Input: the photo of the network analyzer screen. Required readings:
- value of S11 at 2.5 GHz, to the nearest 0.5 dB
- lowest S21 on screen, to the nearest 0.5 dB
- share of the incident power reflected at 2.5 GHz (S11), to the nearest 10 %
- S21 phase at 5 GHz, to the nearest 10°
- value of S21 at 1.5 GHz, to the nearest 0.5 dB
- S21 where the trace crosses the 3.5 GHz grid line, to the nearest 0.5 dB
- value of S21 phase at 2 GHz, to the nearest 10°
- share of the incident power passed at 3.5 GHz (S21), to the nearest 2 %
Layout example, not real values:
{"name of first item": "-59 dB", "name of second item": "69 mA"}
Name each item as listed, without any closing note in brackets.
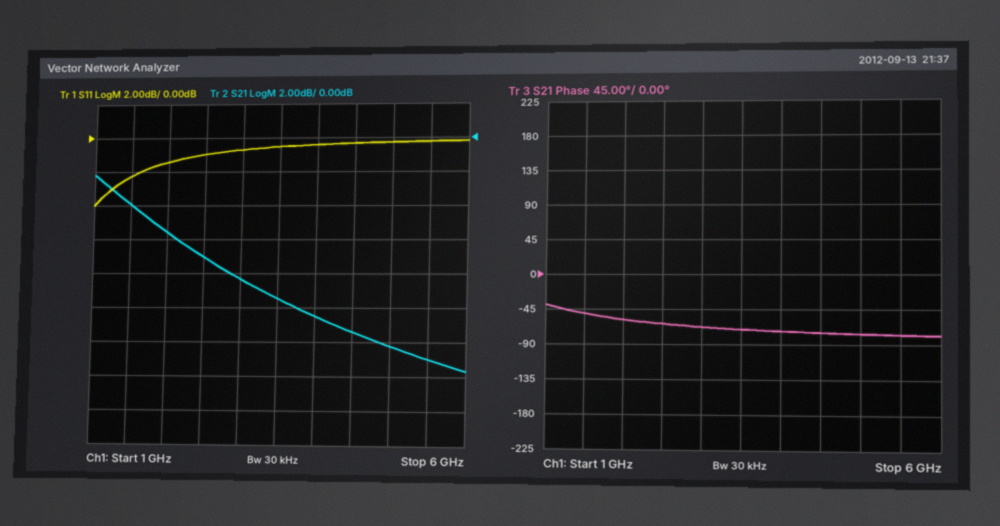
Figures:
{"value of S11 at 2.5 GHz, to the nearest 0.5 dB": "-1.0 dB", "lowest S21 on screen, to the nearest 0.5 dB": "-13.5 dB", "share of the incident power reflected at 2.5 GHz (S11), to the nearest 10 %": "80 %", "S21 phase at 5 GHz, to the nearest 10°": "-80°", "value of S21 at 1.5 GHz, to the nearest 0.5 dB": "-4.0 dB", "S21 where the trace crosses the 3.5 GHz grid line, to the nearest 0.5 dB": "-9.5 dB", "value of S21 phase at 2 GHz, to the nearest 10°": "-60°", "share of the incident power passed at 3.5 GHz (S21), to the nearest 2 %": "12 %"}
